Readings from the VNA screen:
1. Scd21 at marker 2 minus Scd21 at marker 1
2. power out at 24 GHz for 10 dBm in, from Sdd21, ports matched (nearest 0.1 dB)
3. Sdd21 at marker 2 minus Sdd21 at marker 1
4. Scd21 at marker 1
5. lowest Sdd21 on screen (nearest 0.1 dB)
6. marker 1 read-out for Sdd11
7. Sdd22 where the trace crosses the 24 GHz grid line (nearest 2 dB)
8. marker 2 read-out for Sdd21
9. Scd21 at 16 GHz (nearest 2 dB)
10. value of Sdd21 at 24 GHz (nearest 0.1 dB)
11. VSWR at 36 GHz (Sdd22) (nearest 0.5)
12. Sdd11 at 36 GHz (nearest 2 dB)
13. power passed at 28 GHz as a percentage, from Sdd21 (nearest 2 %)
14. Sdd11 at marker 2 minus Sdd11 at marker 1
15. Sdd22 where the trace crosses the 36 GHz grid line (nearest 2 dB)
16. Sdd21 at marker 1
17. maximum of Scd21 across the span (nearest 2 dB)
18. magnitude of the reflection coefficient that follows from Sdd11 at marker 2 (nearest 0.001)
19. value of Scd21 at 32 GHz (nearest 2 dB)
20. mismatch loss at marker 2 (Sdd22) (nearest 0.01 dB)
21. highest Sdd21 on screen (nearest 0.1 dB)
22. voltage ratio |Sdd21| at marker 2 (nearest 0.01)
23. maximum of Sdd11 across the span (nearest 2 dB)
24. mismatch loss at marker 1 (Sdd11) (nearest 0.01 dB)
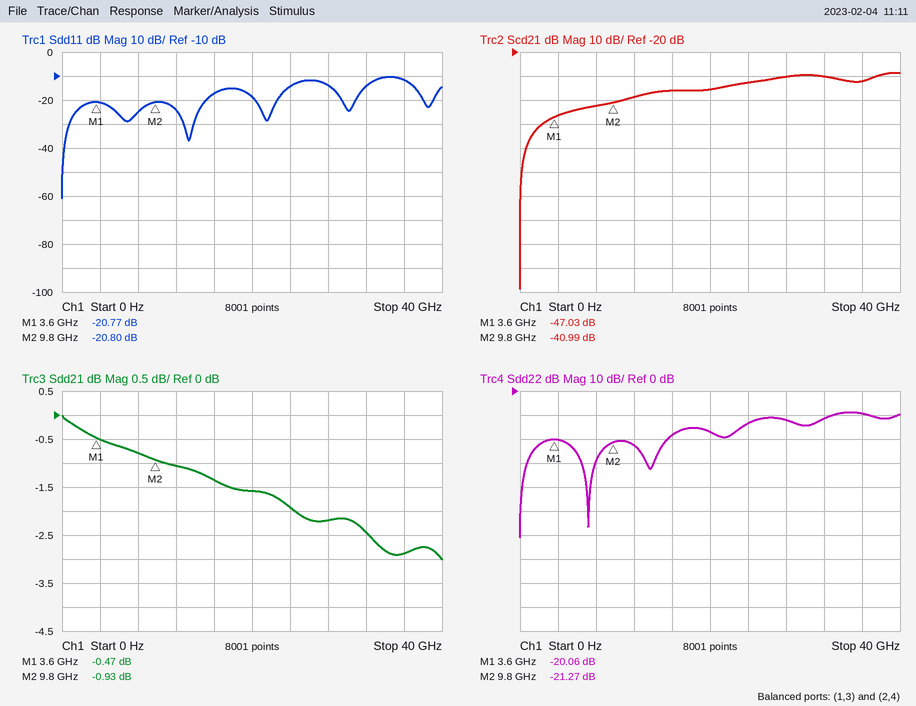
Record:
6.04 dB
8.1 dBm
-0.46 dB
-47.03 dB
-3.0 dB
-20.77 dB
-14 dB
-0.93 dB
-36 dB
-1.9 dB
2.0
-12 dB
60 %
-0.03 dB
-10 dB
-0.47 dB
-28 dB
0.091
-30 dB
0.03 dB
0.0 dB
0.90
-10 dB
0.04 dB
